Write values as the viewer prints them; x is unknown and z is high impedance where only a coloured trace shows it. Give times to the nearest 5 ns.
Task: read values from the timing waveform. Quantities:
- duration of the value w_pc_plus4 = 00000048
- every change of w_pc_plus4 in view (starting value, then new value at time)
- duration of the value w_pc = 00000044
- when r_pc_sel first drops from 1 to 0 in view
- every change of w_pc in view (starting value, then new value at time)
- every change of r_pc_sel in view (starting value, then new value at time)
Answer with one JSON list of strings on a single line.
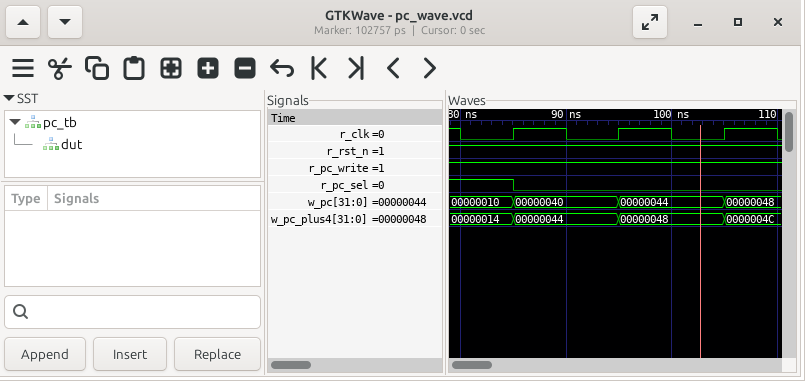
["10 ns", "00000014, 00000044 at 85 ns, 00000048 at 95 ns, 0000004C at 105 ns", "10 ns", "85 ns", "00000010, 00000040 at 85 ns, 00000044 at 95 ns, 00000048 at 105 ns", "1, 0 at 85 ns"]
